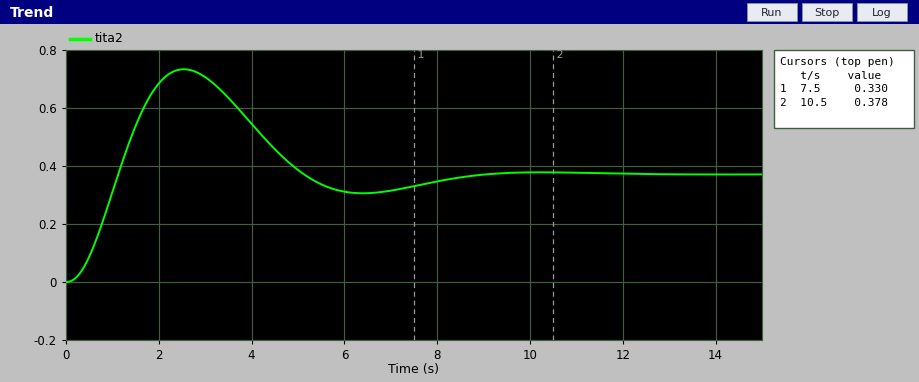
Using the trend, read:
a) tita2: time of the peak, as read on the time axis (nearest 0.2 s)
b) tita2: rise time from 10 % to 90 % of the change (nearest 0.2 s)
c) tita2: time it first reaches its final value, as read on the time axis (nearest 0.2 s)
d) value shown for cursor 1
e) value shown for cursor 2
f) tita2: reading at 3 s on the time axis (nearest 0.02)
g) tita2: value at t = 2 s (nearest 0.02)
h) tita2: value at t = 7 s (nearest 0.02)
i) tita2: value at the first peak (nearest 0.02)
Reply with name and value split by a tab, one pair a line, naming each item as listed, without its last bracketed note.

tita2: time of the peak, as read on the time axis	2.6 s
tita2: rise time from 10 % to 90 % of the change	0.8 s
tita2: time it first reaches its final value, as read on the time axis	1.2 s
value shown for cursor 1	0.330
value shown for cursor 2	0.378
tita2: reading at 3 s on the time axis	0.70
tita2: value at t = 2 s	0.68
tita2: value at t = 7 s	0.32
tita2: value at the first peak	0.74
